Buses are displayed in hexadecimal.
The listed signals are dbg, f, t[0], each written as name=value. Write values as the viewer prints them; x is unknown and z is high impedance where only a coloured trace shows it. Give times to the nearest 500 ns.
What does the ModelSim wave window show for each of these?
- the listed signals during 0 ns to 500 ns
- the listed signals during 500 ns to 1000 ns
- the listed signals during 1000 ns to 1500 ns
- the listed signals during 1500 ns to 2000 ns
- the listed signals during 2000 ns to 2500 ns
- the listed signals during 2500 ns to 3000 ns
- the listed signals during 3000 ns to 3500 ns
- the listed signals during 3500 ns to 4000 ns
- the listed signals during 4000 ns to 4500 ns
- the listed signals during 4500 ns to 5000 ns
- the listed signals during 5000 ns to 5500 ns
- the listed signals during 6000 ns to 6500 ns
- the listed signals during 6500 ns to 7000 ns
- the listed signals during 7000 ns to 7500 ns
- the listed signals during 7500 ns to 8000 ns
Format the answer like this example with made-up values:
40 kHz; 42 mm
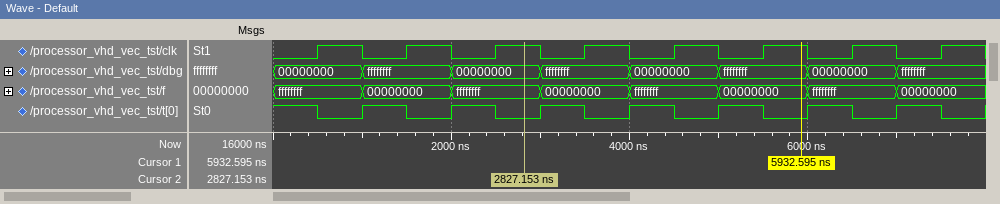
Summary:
dbg=00000000, f=ffffffff, t[0]=1; dbg=00000000, f=ffffffff, t[0]=0; dbg=ffffffff, f=00000000, t[0]=1; dbg=ffffffff, f=00000000, t[0]=0; dbg=00000000, f=ffffffff, t[0]=1; dbg=00000000, f=ffffffff, t[0]=0; dbg=ffffffff, f=00000000, t[0]=1; dbg=ffffffff, f=00000000, t[0]=0; dbg=00000000, f=ffffffff, t[0]=1; dbg=00000000, f=ffffffff, t[0]=0; dbg=ffffffff, f=00000000, t[0]=1; dbg=00000000, f=ffffffff, t[0]=1; dbg=00000000, f=ffffffff, t[0]=0; dbg=ffffffff, f=00000000, t[0]=1; dbg=ffffffff, f=00000000, t[0]=0
